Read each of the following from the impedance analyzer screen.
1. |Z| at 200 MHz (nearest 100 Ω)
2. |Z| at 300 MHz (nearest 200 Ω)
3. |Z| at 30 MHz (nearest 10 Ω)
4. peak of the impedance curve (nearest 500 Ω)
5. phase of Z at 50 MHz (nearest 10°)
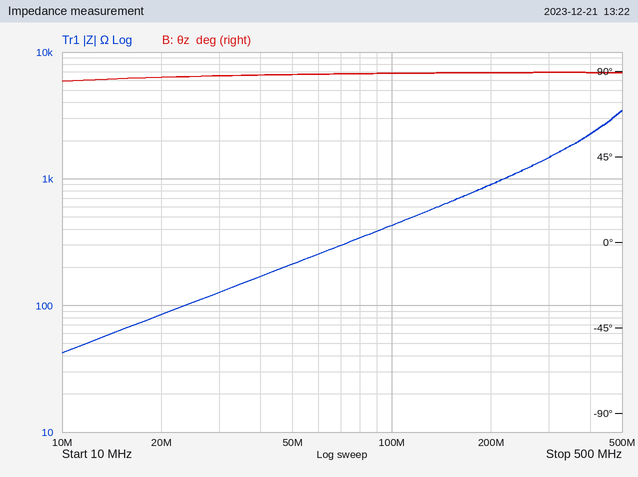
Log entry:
900 Ω
1.4 kΩ
130 Ω
3.5 kΩ
90°
